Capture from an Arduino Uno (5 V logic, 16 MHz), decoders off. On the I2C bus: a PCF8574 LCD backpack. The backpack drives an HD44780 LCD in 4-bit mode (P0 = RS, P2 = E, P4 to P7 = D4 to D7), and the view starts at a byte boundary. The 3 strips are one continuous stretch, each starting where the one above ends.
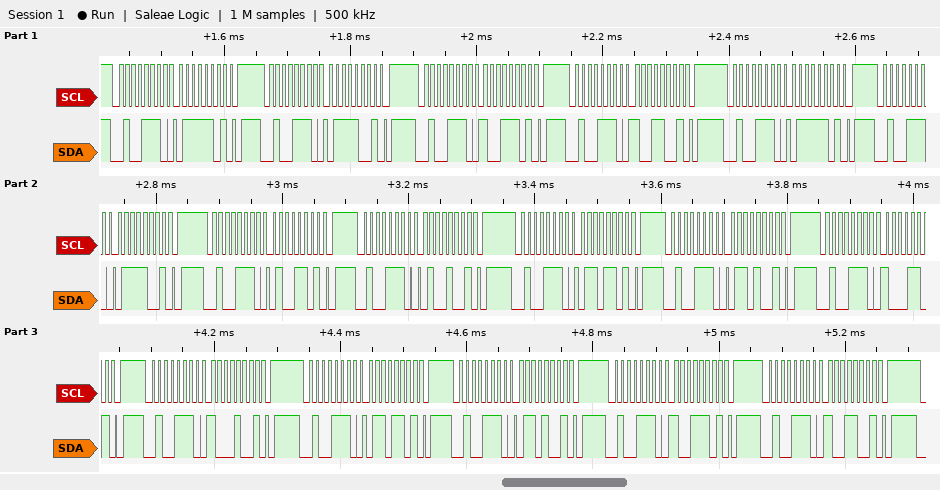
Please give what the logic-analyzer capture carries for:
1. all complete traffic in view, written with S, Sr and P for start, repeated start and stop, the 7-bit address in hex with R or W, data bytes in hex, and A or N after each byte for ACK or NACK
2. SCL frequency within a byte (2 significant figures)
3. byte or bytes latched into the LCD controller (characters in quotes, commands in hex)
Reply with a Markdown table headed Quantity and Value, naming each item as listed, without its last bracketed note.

| Quantity | Value |
|---|---|
| all complete traffic in view, written with S, Sr and P for start, repeated start and stop, the 7-bit address in hex with R or W, data bytes in hex, and A or N after each byte for ACK or NACK | S 27W A 7D A P S 27W A 79 A P S 27W A 9D A P S 27W A 99 A P S 27W A 7D A P S 27W A 79 A P S 27W A 4D A P S 27W A 49 A P S 27W A 6D A P S 27W A 69 A P S 27W A 8D A P S 27W A 89 A P S 27W A 6D A P S 27W A 69 A P S 27W A 9D A P S 27W A 99 A P |
| SCL frequency within a byte | 100 kHz |
| byte or bytes latched into the LCD controller | 'y' 't' 'h' 'i' |
